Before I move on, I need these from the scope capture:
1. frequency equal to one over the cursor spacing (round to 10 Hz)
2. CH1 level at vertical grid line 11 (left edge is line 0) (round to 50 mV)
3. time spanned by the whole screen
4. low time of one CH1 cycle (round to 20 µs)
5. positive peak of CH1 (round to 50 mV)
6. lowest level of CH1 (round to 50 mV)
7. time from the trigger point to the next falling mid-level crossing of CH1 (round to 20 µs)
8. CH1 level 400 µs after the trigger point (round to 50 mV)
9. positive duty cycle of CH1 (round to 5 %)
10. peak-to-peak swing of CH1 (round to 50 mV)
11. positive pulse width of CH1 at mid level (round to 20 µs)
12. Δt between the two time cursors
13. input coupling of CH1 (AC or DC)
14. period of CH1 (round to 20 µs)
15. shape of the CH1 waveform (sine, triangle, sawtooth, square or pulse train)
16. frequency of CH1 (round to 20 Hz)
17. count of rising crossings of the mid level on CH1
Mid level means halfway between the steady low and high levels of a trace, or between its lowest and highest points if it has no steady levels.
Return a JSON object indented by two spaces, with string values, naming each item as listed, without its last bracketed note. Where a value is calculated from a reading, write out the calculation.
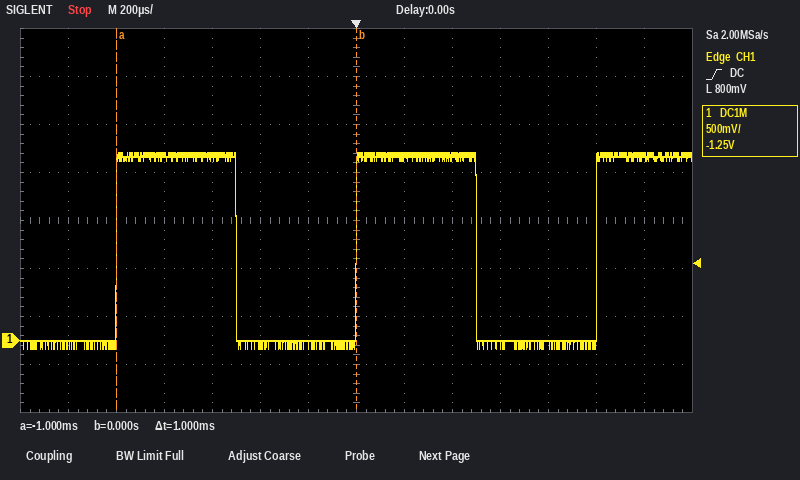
{
  "frequency equal to one over the cursor spacing": "1 / 1 ms ≈ 1.00 kHz",
  "CH1 level at vertical grid line 11 (left edge is line 0)": "-50 mV",
  "time spanned by the whole screen": "2.8 ms",
  "low time of one CH1 cycle": "500 µs",
  "positive peak of CH1": "1.95 V",
  "lowest level of CH1": "-100 mV",
  "time from the trigger point to the next falling mid-level crossing of CH1": "500 µs",
  "CH1 level 400 µs after the trigger point": "1.90 V",
  "positive duty cycle of CH1": "500 µs / 1.00 ms ≈ 50 %",
  "peak-to-peak swing of CH1": "1.95 V − (-100 mV) = 2.05 V",
  "positive pulse width of CH1 at mid level": "500 µs",
  "Δt between the two time cursors": "1 ms",
  "input coupling of CH1": "DC",
  "period of CH1": "1.00 ms",
  "shape of the CH1 waveform": "square",
  "frequency of CH1": "1 / 1.00 ms ≈ 1.00 kHz",
  "count of rising crossings of the mid level on CH1": "3"
}
